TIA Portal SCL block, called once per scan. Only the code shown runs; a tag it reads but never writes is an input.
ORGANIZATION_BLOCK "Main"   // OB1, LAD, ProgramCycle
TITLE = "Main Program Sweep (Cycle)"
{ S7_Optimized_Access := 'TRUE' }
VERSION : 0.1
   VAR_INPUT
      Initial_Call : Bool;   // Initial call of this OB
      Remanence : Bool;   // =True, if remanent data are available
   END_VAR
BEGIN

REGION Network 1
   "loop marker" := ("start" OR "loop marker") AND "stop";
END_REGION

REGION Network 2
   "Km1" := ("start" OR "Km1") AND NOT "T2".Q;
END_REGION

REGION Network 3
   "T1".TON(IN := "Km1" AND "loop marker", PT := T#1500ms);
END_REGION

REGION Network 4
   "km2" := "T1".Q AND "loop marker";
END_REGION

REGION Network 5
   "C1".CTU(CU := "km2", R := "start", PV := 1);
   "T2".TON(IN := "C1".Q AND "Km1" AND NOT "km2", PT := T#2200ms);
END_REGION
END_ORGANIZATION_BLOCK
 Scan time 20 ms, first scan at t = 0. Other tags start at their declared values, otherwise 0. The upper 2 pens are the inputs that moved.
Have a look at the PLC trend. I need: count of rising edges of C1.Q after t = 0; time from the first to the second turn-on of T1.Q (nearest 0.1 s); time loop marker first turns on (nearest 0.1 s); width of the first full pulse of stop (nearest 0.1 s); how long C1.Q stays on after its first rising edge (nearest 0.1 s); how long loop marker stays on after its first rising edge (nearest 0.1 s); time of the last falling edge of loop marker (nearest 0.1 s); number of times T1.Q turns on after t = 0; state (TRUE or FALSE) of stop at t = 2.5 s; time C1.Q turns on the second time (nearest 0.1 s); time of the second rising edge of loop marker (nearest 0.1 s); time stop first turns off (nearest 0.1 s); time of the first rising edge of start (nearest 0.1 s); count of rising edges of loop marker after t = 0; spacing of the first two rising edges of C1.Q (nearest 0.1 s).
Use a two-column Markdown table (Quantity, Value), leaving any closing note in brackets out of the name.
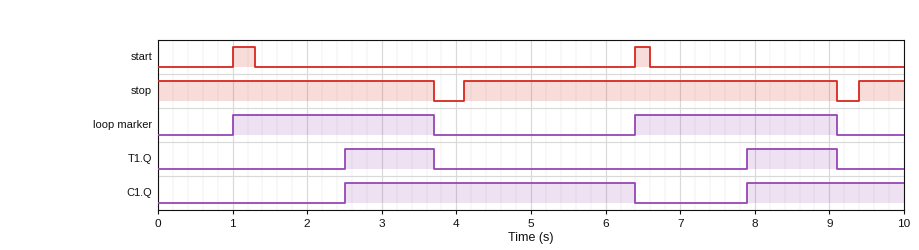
| Quantity | Value |
|---|---|
| count of rising edges of C1.Q after t = 0 | 2 |
| time from the first to the second turn-on of T1.Q | 5.4 s |
| time loop marker first turns on | 1.0 s |
| width of the first full pulse of stop | 5.0 s |
| how long C1.Q stays on after its first rising edge | 3.9 s |
| how long loop marker stays on after its first rising edge | 2.7 s |
| time of the last falling edge of loop marker | 9.1 s |
| number of times T1.Q turns on after t = 0 | 2 |
| state (TRUE or FALSE) of stop at t = 2.5 s | TRUE |
| time C1.Q turns on the second time | 7.9 s |
| time of the second rising edge of loop marker | 6.4 s |
| time stop first turns off | 3.7 s |
| time of the first rising edge of start | 1.0 s |
| count of rising edges of loop marker after t = 0 | 2 |
| spacing of the first two rising edges of C1.Q | 5.4 s |
